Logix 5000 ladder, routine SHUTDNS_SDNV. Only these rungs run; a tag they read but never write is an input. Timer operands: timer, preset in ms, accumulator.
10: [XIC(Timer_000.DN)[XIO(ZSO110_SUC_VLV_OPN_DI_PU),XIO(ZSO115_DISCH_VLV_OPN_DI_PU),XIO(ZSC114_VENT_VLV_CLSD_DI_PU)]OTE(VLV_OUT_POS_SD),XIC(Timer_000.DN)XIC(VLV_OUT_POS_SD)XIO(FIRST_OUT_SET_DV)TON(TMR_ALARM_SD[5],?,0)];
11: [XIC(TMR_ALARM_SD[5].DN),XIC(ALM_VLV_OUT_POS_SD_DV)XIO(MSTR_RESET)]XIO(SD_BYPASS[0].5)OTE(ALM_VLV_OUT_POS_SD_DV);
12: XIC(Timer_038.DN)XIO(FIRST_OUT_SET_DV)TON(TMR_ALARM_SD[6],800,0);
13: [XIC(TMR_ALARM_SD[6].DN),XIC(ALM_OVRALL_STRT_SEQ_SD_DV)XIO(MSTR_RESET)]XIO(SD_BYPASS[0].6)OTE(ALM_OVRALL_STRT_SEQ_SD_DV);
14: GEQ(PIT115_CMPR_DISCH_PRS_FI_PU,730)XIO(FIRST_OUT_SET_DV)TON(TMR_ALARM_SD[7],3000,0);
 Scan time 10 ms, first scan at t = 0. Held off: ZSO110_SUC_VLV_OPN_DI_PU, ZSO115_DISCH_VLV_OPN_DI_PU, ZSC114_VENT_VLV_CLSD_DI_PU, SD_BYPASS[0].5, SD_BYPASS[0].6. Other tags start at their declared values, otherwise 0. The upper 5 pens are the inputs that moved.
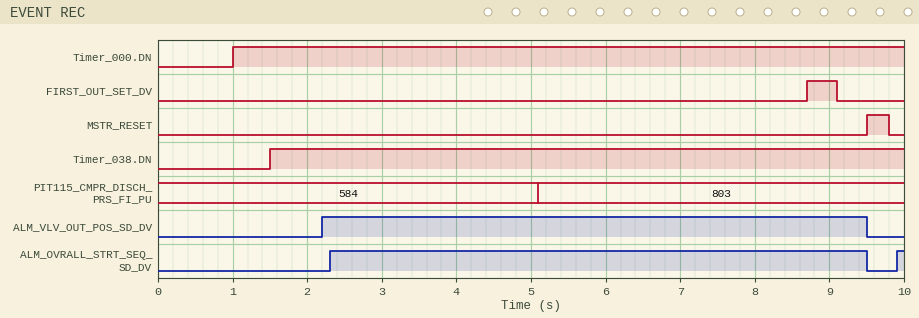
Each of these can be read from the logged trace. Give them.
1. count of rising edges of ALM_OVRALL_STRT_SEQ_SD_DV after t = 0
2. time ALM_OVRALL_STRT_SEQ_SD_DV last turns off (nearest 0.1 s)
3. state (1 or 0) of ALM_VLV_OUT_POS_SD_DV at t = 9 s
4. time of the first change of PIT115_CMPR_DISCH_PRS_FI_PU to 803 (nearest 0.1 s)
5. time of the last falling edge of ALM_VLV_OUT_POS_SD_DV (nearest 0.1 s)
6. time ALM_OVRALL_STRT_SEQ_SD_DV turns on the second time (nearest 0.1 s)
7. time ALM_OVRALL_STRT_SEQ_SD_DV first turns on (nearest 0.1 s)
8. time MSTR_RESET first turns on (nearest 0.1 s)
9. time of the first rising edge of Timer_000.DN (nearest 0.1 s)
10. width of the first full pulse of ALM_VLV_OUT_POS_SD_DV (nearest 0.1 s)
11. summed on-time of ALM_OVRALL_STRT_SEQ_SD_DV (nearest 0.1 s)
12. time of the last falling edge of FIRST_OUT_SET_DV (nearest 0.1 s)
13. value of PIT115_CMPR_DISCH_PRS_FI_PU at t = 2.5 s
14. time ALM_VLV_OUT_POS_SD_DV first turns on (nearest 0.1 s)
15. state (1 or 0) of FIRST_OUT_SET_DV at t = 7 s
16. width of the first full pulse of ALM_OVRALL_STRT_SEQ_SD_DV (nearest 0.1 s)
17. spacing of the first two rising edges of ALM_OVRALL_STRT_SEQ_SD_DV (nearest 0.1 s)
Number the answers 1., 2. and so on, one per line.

1. 2
2. 9.5 s
3. 1
4. 5.1 s
5. 9.5 s
6. 9.9 s
7. 2.3 s
8. 9.5 s
9. 1.0 s
10. 7.3 s
11. 7.3 s
12. 9.1 s
13. 584
14. 2.2 s
15. 0
16. 7.2 s
17. 7.6 s
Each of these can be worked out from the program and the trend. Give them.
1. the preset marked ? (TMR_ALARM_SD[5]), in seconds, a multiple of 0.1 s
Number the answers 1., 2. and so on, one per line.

1. 1.2 s
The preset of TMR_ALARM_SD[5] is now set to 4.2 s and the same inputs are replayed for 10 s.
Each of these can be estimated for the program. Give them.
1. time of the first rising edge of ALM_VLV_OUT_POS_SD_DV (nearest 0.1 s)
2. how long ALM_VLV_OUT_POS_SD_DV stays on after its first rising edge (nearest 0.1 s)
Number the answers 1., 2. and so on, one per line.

1. 5.2 s
2. 4.3 s
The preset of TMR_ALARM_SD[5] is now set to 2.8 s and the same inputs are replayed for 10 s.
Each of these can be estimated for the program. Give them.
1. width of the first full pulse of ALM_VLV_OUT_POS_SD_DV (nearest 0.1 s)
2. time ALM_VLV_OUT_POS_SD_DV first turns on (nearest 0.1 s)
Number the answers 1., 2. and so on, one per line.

1. 5.7 s
2. 3.8 s
